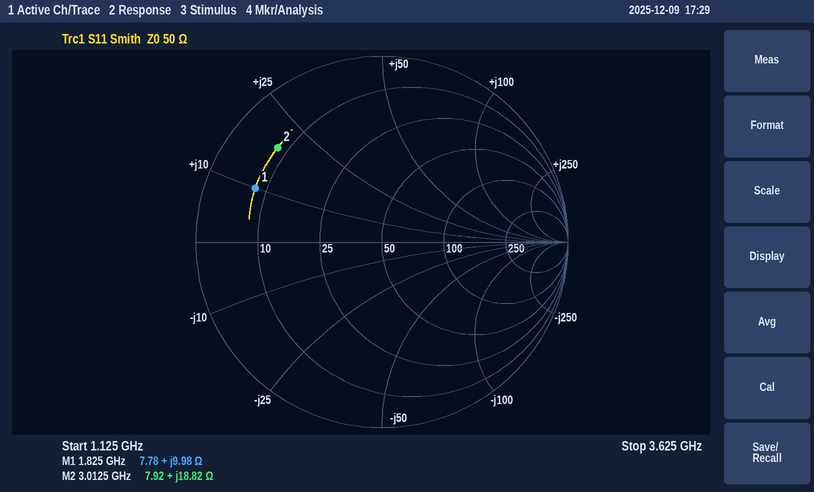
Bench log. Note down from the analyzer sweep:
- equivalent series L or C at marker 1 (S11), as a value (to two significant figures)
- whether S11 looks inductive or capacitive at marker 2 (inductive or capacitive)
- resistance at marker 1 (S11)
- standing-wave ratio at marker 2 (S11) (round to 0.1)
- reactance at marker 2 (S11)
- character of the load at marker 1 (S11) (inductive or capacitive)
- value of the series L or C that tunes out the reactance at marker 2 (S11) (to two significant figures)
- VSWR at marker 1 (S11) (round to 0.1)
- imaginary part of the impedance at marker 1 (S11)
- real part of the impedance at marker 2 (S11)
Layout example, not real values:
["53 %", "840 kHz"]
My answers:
["870 pH", "inductive", "7.78 Ω", "7.2", "+18.82 Ω", "inductive", "2.8 pF", "6.7", "+9.98 Ω", "7.92 Ω"]
